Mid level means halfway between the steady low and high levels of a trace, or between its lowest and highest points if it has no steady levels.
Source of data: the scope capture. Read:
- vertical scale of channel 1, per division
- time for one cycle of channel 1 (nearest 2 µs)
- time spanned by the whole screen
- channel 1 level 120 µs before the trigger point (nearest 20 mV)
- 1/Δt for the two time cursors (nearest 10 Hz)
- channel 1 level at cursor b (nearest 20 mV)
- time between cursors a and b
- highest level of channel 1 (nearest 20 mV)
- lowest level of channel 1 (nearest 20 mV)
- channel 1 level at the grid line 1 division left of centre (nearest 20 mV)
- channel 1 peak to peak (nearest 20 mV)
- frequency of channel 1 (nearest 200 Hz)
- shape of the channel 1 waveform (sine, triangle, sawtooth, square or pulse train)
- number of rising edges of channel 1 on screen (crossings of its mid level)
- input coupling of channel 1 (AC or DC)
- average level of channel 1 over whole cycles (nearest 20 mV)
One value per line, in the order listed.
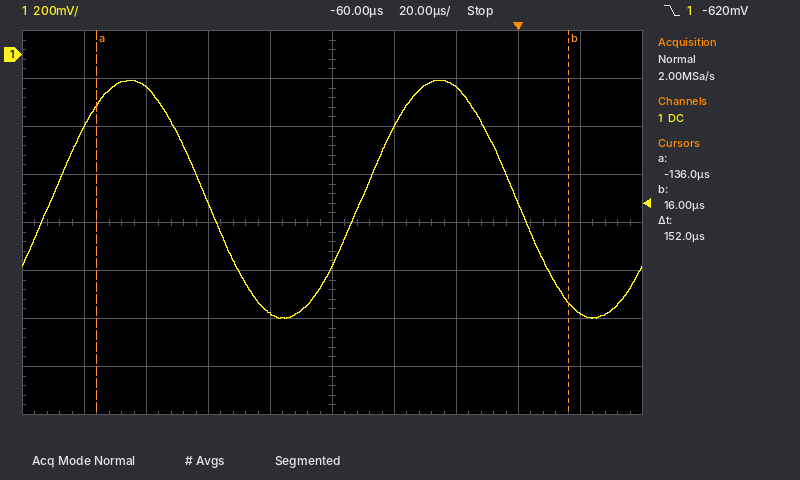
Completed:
200 mV
100 µs
200 µs
-140 mV
6.58 kHz
-1.04 V
152 µs
-100 mV
-1.10 V
-1.08 V
1.00 V
10.0 kHz
sine
2
DC
-600 mV
